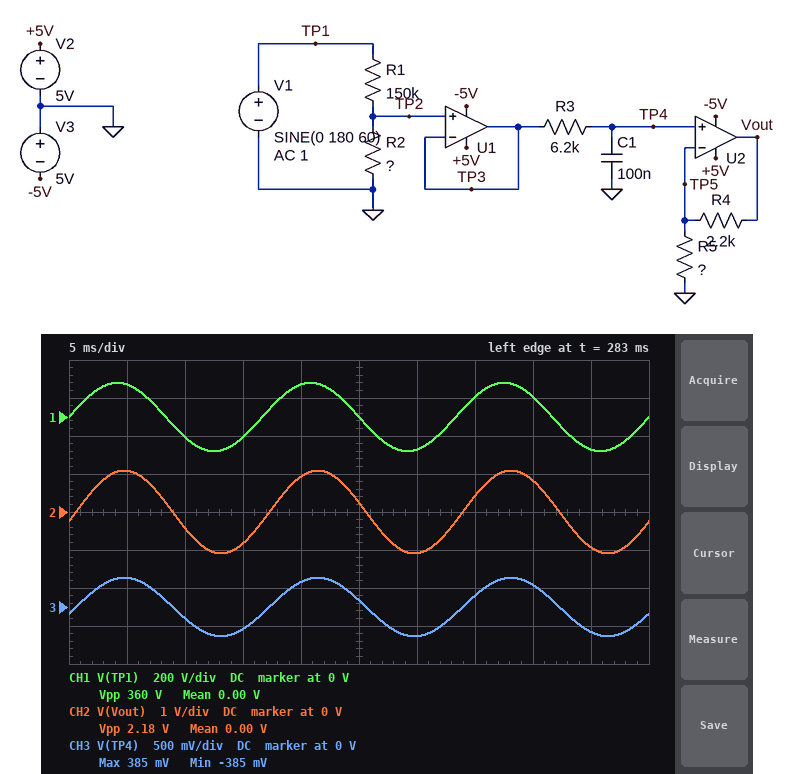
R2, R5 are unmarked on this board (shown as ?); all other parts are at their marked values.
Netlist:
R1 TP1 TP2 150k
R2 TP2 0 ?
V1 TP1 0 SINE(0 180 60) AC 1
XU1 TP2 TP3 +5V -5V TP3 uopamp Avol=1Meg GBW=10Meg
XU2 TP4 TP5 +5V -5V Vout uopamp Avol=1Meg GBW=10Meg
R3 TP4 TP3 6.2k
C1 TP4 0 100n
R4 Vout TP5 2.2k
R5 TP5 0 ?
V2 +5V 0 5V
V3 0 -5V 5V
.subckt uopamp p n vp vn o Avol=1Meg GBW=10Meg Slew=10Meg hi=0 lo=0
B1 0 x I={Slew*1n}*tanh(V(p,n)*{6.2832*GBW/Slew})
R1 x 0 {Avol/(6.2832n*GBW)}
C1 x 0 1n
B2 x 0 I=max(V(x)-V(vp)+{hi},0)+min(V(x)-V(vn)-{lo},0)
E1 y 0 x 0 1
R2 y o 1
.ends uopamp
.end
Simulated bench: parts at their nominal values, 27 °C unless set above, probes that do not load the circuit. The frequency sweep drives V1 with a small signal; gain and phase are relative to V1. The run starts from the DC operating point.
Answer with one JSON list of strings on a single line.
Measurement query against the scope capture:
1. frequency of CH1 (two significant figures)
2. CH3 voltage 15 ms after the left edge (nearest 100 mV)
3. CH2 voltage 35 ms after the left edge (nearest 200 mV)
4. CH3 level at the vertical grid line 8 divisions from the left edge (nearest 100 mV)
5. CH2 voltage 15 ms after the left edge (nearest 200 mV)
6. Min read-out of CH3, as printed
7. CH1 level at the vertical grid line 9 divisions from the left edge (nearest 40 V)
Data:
["60 Hz", "-300 mV", "400 mV", "300 mV", "-800 mV", "-385 mV", "-160 V"]
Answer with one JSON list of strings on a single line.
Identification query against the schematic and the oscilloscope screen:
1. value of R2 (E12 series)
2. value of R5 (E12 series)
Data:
["330 Ω", "1.2 kΩ"]
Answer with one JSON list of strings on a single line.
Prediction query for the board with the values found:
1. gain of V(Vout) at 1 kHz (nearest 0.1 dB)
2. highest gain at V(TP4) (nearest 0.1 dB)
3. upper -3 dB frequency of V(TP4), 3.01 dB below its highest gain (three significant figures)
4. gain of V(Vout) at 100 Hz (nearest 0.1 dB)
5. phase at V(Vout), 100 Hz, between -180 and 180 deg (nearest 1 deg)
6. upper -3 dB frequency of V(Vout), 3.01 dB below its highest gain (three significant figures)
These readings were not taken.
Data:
["-56.2 dB", "-53.2 dB", "257 Hz", "-44.7 dB", "-21 deg", "257 Hz"]
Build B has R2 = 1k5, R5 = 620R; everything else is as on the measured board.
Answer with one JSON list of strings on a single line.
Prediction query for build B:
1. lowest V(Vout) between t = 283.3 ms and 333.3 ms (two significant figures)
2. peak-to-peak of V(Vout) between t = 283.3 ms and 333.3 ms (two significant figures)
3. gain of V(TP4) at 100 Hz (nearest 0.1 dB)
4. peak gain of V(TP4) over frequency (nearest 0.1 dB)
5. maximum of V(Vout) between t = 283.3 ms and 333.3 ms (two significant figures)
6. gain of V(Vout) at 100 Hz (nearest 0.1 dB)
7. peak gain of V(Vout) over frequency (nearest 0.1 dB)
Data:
["-5.0 V", "10 V", "-40.7 dB", "-40.1 dB", "5.0 V", "-27.5 dB", "-26.9 dB"]
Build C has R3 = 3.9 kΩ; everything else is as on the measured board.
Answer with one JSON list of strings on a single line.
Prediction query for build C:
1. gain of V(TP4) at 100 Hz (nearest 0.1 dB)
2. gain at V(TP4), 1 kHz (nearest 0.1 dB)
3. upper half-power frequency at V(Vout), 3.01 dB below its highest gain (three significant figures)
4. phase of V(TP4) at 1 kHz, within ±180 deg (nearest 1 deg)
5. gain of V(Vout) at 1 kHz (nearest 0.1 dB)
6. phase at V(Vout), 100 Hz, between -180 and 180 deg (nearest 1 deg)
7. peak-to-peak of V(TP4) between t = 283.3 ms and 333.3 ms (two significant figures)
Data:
["-53.4 dB", "-61.6 dB", "408 Hz", "-68 deg", "-52.6 dB", "-14 deg", "780 mV"]
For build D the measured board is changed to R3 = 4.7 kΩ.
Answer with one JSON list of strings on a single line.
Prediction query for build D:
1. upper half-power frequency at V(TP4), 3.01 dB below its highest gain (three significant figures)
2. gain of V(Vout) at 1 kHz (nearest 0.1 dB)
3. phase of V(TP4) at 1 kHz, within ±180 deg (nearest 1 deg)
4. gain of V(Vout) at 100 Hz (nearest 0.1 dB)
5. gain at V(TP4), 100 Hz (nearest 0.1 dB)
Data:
["339 Hz", "-54.0 dB", "-71 deg", "-44.5 dB", "-53.5 dB"]
